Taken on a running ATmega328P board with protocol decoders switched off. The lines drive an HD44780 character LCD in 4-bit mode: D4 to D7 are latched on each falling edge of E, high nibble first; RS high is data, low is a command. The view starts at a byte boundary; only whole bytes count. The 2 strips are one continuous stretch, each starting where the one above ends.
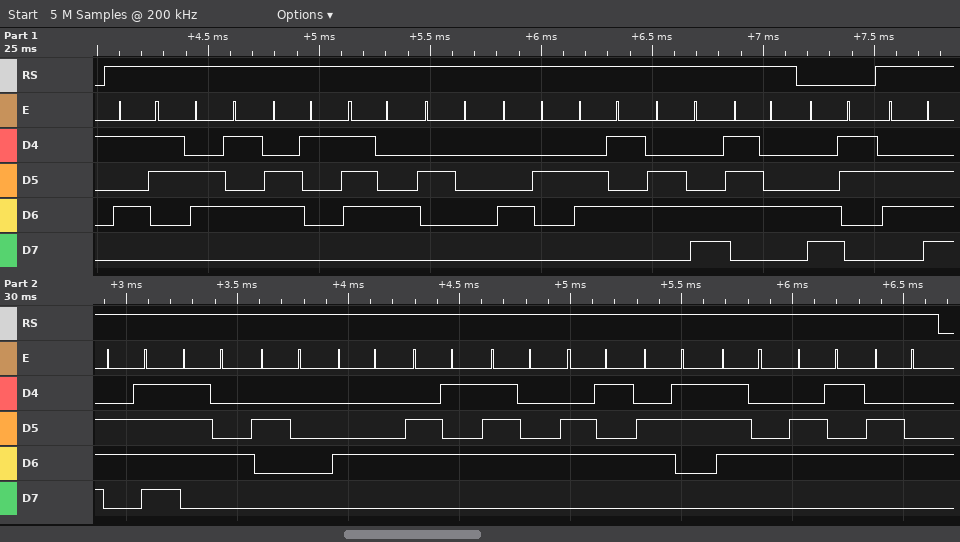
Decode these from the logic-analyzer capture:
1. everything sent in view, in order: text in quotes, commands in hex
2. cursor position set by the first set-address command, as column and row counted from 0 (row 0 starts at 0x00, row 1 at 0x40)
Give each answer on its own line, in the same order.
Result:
"Seat Belt" 0xC3 "not Detected"
column 3, row 1
